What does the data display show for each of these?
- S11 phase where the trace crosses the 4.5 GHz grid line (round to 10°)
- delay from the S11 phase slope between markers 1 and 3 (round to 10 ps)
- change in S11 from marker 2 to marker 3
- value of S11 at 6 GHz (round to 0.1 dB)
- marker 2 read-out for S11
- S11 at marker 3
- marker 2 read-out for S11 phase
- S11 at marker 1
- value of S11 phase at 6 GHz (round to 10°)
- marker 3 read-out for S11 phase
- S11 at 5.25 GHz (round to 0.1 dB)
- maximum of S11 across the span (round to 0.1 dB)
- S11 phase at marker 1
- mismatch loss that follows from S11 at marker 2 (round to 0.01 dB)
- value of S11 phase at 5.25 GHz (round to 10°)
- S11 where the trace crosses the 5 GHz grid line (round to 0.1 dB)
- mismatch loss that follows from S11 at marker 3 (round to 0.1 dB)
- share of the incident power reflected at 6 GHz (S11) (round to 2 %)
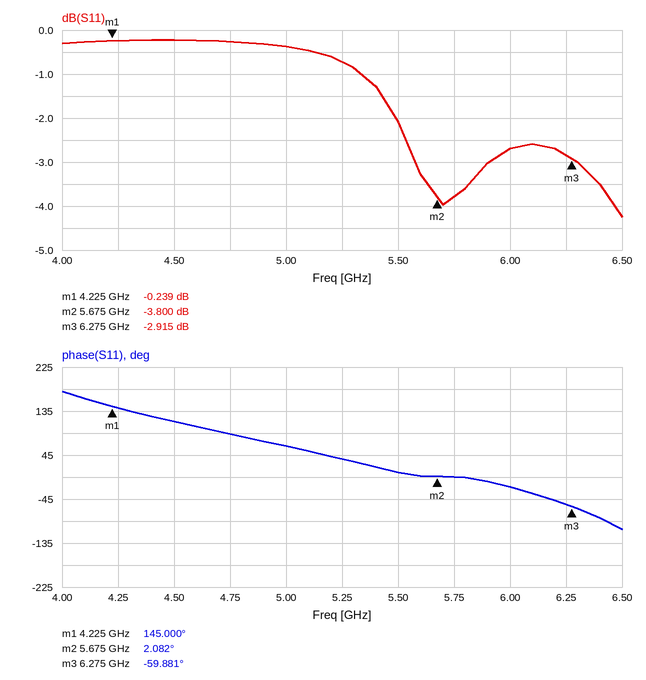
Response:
110°
280 ps
0.885 dB
-2.7 dB
-3.800 dB
-2.915 dB
2.082°
-0.239 dB
-20°
-59.881°
-0.7 dB
-0.2 dB
145.000°
2.34 dB
40°
-0.4 dB
3.1 dB
54 %
